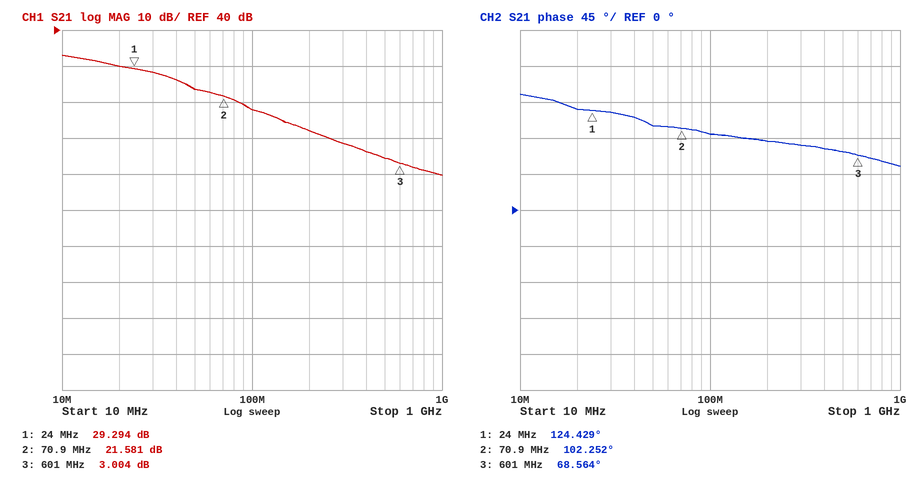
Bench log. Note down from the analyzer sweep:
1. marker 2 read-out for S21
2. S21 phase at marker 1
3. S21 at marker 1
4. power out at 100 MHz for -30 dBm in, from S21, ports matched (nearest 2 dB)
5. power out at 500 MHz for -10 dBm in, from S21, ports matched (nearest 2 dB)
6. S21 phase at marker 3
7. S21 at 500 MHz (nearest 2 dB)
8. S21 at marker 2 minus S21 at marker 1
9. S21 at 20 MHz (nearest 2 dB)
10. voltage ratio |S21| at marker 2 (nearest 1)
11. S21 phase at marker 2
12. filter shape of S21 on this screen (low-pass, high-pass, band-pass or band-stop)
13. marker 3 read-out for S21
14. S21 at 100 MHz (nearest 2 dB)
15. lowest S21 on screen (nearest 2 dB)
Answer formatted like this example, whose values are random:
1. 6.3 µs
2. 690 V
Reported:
1. 21.581 dB
2. 124.429°
3. 29.294 dB
4. -12 dBm
5. -6 dBm
6. 68.564°
7. 4 dB
8. -7.713 dB
9. 30 dB
10. 12
11. 102.252°
12. low-pass
13. 3.004 dB
14. 18 dB
15. 0 dB
